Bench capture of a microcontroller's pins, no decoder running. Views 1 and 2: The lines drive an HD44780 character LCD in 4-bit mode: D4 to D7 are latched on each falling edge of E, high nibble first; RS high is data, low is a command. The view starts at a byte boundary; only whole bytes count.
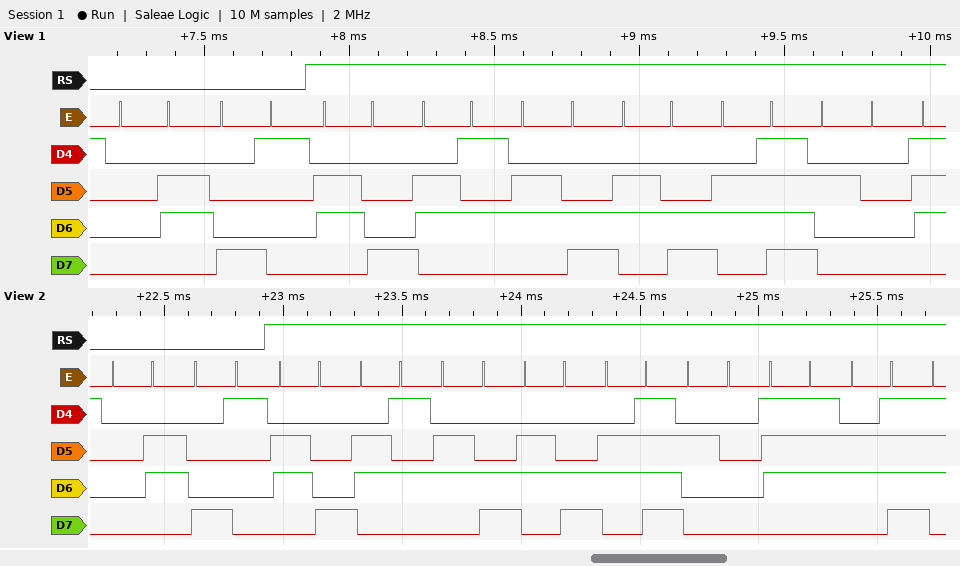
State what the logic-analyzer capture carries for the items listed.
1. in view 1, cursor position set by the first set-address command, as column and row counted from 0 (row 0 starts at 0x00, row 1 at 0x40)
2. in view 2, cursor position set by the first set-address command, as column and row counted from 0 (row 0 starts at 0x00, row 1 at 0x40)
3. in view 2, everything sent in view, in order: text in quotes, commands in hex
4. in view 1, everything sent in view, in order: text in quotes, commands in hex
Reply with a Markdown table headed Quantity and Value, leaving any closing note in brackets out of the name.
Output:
| Quantity | Value |
|---|---|
| in view 1, cursor position set by the first set-address command, as column and row counted from 0 | column 1, row 0 |
| in view 2, cursor position set by the first set-address command, as column and row counted from 0 | column 1, row 0 |
| in view 2, everything sent in view, in order: text in quotes, commands in hex | 0x06 0x81 "hello wo" |
| in view 1, everything sent in view, in order: text in quotes, commands in hex | 0x06 0x81 "hello " |
